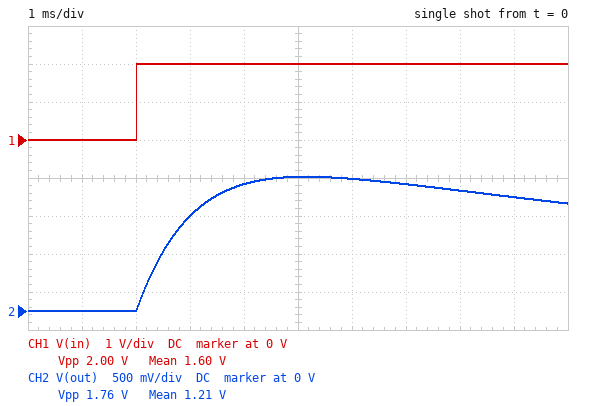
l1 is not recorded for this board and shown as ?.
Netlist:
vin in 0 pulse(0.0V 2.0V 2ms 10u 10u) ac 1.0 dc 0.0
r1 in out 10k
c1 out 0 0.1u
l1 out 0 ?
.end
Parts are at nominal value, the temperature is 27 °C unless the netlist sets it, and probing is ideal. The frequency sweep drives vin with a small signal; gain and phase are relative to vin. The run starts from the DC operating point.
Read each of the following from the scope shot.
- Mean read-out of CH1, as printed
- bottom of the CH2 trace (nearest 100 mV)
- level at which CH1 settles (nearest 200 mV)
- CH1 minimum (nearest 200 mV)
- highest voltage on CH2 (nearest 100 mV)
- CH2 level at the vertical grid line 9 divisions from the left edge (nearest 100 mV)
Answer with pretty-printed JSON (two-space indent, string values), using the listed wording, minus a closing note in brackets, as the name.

{
  "Mean read-out of CH1, as printed": "1.60 V",
  "bottom of the CH2 trace": "0 V",
  "level at which CH1 settles": "2.0 V",
  "CH1 minimum": "0 V",
  "highest voltage on CH2": "1.8 V",
  "CH2 level at the vertical grid line 9 divisions from the left edge": "1.5 V"
}
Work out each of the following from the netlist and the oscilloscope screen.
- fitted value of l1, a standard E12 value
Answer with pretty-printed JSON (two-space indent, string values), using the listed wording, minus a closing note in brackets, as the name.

{
  "fitted value of l1, a standard E12 value": "180 H"
}
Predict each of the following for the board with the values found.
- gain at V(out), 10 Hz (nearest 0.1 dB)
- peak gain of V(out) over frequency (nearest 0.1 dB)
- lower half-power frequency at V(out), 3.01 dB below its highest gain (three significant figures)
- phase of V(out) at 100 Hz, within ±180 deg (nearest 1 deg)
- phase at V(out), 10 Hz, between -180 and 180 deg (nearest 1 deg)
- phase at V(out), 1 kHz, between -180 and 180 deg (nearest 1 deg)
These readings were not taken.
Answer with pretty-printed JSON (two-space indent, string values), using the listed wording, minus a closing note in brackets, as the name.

{
  "gain at V(out), 10 Hz": "-2.2 dB",
  "peak gain of V(out) over frequency": "0 dB",
  "lower half-power frequency at V(out), 3.01 dB below its highest gain": "8.40 Hz",
  "phase of V(out) at 100 Hz, within ±180 deg": "-28 deg",
  "phase at V(out), 10 Hz, between -180 and 180 deg": "39 deg",
  "phase at V(out), 1 kHz, between -180 and 180 deg": "-81 deg"
}
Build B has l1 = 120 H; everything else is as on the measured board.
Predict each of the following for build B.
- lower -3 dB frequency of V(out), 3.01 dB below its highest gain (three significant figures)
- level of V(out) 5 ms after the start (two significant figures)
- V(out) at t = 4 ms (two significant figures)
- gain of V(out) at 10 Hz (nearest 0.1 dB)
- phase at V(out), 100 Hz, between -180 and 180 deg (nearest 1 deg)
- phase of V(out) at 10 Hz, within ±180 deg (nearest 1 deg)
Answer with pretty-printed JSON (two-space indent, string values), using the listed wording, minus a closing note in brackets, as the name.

{
  "lower -3 dB frequency of V(out), 3.01 dB below its highest gain": "12.3 Hz",
  "level of V(out) 5 ms after the start": "1.7 V",
  "V(out) at t = 4 ms": "1.6 V",
  "gain of V(out) at 10 Hz": "-4.1 dB",
  "phase at V(out), 100 Hz, between -180 and 180 deg": "-26 deg",
  "phase of V(out) at 10 Hz, within ±180 deg": "52 deg"
}
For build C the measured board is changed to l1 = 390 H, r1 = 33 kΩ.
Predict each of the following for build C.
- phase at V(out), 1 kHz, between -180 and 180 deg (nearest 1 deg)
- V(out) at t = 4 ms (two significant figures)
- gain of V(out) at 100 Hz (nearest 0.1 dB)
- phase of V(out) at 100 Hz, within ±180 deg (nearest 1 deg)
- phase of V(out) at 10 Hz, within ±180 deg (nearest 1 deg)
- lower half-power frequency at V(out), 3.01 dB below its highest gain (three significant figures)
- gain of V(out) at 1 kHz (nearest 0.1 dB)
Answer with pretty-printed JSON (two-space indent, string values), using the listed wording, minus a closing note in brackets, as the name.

{
  "phase at V(out), 1 kHz, between -180 and 180 deg": "-87 deg",
  "V(out) at t = 4 ms": "890 mV",
  "gain of V(out) at 100 Hz": "-6.8 dB",
  "phase of V(out) at 100 Hz, within ±180 deg": "-63 deg",
  "phase of V(out) at 10 Hz, within ±180 deg": "49 deg",
  "lower half-power frequency at V(out), 3.01 dB below its highest gain": "11.0 Hz",
  "gain of V(out) at 1 kHz": "-26.3 dB"
}
